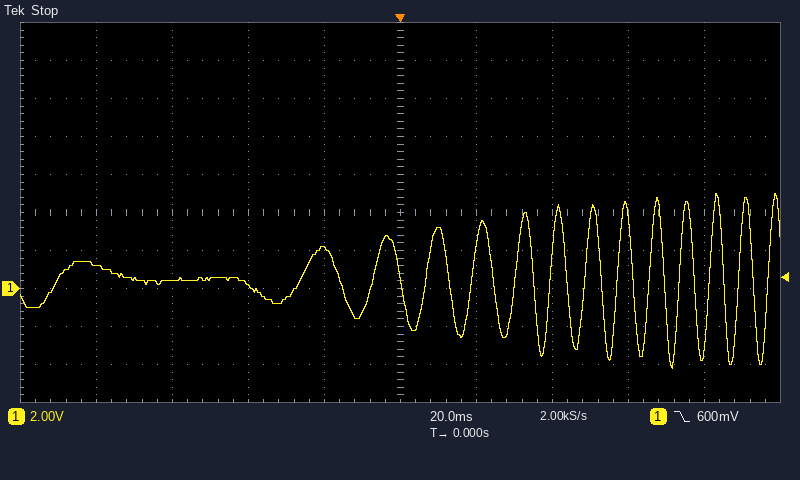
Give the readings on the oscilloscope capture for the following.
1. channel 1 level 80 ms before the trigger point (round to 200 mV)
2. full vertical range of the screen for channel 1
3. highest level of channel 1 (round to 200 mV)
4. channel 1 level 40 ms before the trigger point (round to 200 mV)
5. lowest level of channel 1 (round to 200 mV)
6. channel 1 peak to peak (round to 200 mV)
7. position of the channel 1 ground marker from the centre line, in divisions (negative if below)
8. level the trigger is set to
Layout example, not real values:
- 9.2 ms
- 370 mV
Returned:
- 1.2 V
- 20 V
- 5.0 V
- 200 mV
- -4.2 V
- 9.2 V
- -2.0 div
- 600 mV
